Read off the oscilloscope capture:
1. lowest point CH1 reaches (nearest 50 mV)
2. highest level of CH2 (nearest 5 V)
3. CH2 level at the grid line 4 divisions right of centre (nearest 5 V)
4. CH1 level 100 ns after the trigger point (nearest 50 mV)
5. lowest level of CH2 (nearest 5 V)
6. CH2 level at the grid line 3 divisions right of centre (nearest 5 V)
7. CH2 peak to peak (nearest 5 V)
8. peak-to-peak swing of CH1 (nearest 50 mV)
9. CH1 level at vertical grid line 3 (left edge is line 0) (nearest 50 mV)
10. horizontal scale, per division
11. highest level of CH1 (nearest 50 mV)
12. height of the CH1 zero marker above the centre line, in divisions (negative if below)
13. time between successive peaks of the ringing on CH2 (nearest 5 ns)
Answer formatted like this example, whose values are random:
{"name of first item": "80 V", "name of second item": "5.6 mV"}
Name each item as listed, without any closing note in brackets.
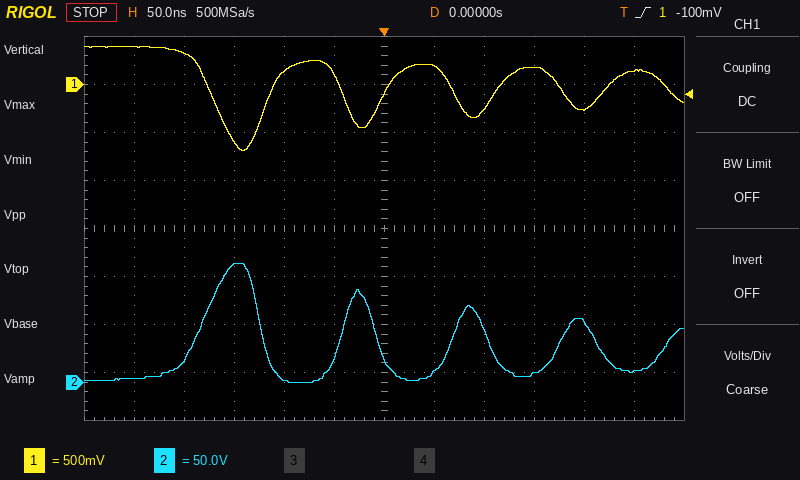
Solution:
{"lowest point CH1 reaches": "-700 mV", "highest level of CH2": "125 V", "CH2 level at the grid line 4 divisions right of centre": "60 V", "CH1 level 100 ns after the trigger point": "-250 mV", "lowest level of CH2": "0 V", "CH2 level at the grid line 3 divisions right of centre": "10 V", "CH2 peak to peak": "125 V", "peak-to-peak swing of CH1": "1.10 V", "CH1 level at vertical grid line 3 (left edge is line 0)": "-600 mV", "horizontal scale, per division": "50 ns", "highest level of CH1": "400 mV", "height of the CH1 zero marker above the centre line, in divisions": "+3.0 div", "time between successive peaks of the ringing on CH2": "115 ns"}
